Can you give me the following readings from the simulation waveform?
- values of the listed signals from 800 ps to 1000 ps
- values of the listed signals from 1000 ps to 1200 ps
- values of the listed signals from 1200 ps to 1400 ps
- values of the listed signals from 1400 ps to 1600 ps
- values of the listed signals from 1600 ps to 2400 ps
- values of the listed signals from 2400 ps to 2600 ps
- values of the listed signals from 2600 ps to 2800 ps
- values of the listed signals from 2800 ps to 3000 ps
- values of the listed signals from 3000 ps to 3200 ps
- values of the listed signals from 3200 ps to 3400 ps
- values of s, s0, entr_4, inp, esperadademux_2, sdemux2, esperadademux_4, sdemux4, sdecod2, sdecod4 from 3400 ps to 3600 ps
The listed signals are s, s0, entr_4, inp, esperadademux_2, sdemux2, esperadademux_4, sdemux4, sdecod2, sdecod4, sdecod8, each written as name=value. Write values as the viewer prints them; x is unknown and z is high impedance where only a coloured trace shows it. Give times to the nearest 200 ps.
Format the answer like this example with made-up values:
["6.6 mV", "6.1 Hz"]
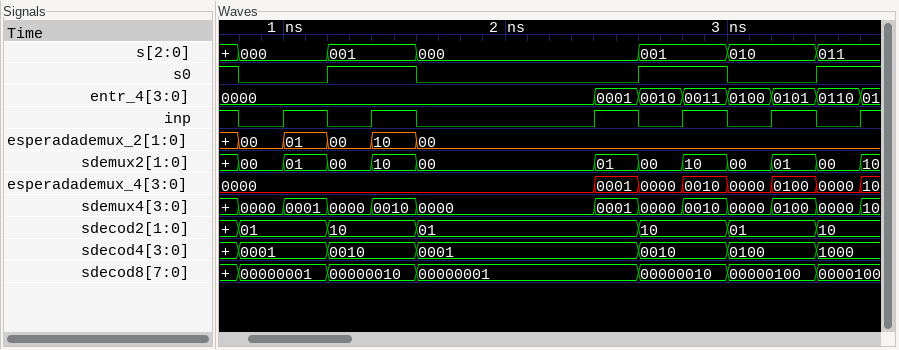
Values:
["s=000, s0=0, entr_4=0000, inp=0, esperadademux_2=00, sdemux2=00, esperadademux_4=0000, sdemux4=0000, sdecod2=01, sdecod4=0001, sdecod8=00000001", "s=000, s0=0, entr_4=0000, inp=1, esperadademux_2=01, sdemux2=01, esperadademux_4=0000, sdemux4=0001, sdecod2=01, sdecod4=0001, sdecod8=00000001", "s=001, s0=1, entr_4=0000, inp=0, esperadademux_2=00, sdemux2=00, esperadademux_4=0000, sdemux4=0000, sdecod2=10, sdecod4=0010, sdecod8=00000010", "s=001, s0=1, entr_4=0000, inp=1, esperadademux_2=10, sdemux2=10, esperadademux_4=0000, sdemux4=0010, sdecod2=10, sdecod4=0010, sdecod8=00000010", "s=000, s0=0, entr_4=0000, inp=0, esperadademux_2=00, sdemux2=00, esperadademux_4=0000, sdemux4=0000, sdecod2=01, sdecod4=0001, sdecod8=00000001", "s=000, s0=0, entr_4=0001, inp=1, esperadademux_2=00, sdemux2=01, esperadademux_4=0001, sdemux4=0001, sdecod2=01, sdecod4=0001, sdecod8=00000001", "s=001, s0=1, entr_4=0010, inp=0, esperadademux_2=00, sdemux2=00, esperadademux_4=0000, sdemux4=0000, sdecod2=10, sdecod4=0010, sdecod8=00000010", "s=001, s0=1, entr_4=0011, inp=1, esperadademux_2=00, sdemux2=10, esperadademux_4=0010, sdemux4=0010, sdecod2=10, sdecod4=0010, sdecod8=00000010", "s=010, s0=0, entr_4=0100, inp=0, esperadademux_2=00, sdemux2=00, esperadademux_4=0000, sdemux4=0000, sdecod2=01, sdecod4=0100, sdecod8=00000100", "s=010, s0=0, entr_4=0101, inp=1, esperadademux_2=00, sdemux2=01, esperadademux_4=0100, sdemux4=0100, sdecod2=01, sdecod4=0100, sdecod8=00000100", "s=011, s0=1, entr_4=0110, inp=0, esperadademux_2=00, sdemux2=00, esperadademux_4=0000, sdemux4=0000, sdecod2=10, sdecod4=1000"]
